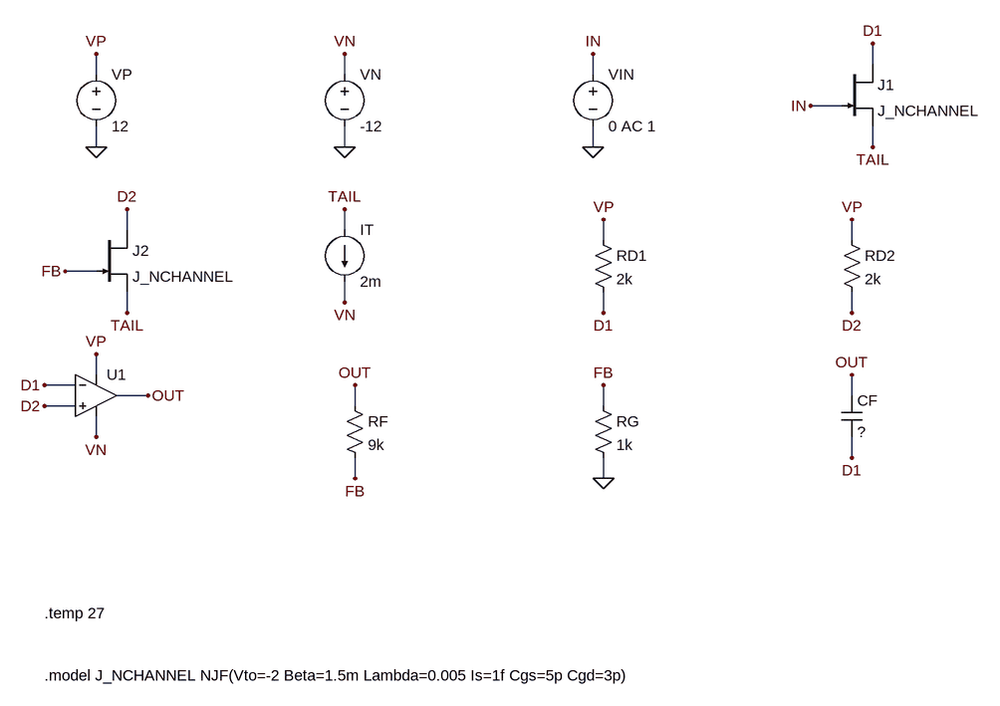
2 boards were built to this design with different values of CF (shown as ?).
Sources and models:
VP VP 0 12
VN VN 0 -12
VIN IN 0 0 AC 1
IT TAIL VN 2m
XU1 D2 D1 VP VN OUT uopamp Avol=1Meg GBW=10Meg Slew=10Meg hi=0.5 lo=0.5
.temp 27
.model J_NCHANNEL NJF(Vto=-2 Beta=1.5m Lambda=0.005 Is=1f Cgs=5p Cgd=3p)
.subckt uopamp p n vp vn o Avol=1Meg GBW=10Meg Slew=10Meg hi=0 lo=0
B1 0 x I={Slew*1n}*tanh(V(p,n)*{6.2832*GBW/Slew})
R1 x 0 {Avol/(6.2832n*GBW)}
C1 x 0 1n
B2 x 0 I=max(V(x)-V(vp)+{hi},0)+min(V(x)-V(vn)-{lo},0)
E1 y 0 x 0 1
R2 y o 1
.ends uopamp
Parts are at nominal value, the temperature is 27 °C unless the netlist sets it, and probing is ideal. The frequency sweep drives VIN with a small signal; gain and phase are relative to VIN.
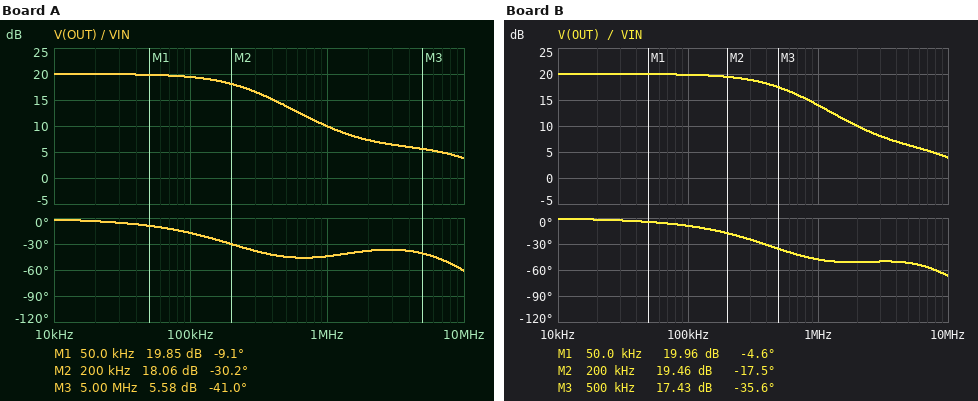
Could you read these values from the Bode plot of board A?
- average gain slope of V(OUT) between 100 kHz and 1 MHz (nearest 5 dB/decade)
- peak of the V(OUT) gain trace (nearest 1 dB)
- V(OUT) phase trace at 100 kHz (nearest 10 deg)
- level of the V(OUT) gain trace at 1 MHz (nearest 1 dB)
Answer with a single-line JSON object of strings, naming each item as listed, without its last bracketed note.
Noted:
{"average gain slope of V(OUT) between 100 kHz and 1 MHz": "-10 dB/decade", "peak of the V(OUT) gain trace": "20 dB", "V(OUT) phase trace at 100 kHz": "-20 deg", "level of the V(OUT) gain trace at 1 MHz": "10 dB"}
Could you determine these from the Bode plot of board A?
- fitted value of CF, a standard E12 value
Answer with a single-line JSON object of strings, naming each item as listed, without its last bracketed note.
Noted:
{"fitted value of CF, a standard E12 value": "120 pF"}
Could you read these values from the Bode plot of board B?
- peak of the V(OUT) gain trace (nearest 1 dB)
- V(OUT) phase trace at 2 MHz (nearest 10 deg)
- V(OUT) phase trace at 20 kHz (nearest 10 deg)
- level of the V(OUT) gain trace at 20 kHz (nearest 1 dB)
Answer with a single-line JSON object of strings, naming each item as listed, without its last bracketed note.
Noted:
{"peak of the V(OUT) gain trace": "20 dB", "V(OUT) phase trace at 2 MHz": "-50 deg", "V(OUT) phase trace at 20 kHz": "0 deg", "level of the V(OUT) gain trace at 20 kHz": "20 dB"}
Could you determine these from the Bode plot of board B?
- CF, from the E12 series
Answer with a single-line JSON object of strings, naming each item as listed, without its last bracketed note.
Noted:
{"CF, from the E12 series": "56 pF"}
